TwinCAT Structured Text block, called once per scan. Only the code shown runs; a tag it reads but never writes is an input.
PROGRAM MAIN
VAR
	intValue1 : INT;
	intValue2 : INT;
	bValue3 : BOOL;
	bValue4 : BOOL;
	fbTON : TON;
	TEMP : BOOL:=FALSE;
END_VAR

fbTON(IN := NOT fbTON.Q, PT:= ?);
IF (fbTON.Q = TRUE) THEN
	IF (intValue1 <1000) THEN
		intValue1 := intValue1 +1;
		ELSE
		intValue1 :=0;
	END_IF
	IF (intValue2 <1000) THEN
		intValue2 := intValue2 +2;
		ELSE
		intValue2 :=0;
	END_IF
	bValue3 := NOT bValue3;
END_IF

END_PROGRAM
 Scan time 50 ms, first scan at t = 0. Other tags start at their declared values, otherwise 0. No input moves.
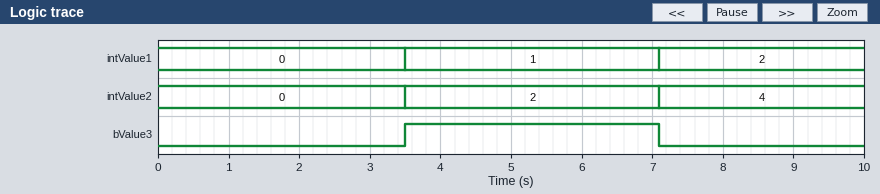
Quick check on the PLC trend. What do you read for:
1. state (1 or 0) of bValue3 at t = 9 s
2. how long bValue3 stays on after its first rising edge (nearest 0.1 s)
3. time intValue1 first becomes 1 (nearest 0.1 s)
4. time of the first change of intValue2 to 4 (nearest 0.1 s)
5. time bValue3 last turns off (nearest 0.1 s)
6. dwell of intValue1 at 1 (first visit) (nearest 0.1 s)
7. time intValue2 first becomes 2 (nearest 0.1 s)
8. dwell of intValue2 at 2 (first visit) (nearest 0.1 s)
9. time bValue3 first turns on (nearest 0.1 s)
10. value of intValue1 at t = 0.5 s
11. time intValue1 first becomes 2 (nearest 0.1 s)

0
3.6 s
3.5 s
7.1 s
7.1 s
3.6 s
3.5 s
3.6 s
3.5 s
0
7.1 s
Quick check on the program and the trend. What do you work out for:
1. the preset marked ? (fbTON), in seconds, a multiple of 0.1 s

3.5 s
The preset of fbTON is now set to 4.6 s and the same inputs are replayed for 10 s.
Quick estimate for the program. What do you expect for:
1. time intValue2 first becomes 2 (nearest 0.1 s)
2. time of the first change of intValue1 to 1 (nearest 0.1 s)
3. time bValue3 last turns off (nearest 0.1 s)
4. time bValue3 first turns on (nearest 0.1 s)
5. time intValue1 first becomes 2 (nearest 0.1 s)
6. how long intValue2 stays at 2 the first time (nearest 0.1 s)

4.6 s
4.6 s
9.3 s
4.6 s
9.3 s
4.7 s
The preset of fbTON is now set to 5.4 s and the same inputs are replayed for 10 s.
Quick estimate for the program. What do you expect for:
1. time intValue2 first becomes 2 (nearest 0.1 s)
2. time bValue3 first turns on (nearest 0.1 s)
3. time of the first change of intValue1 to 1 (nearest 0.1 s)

5.4 s
5.4 s
5.4 s
